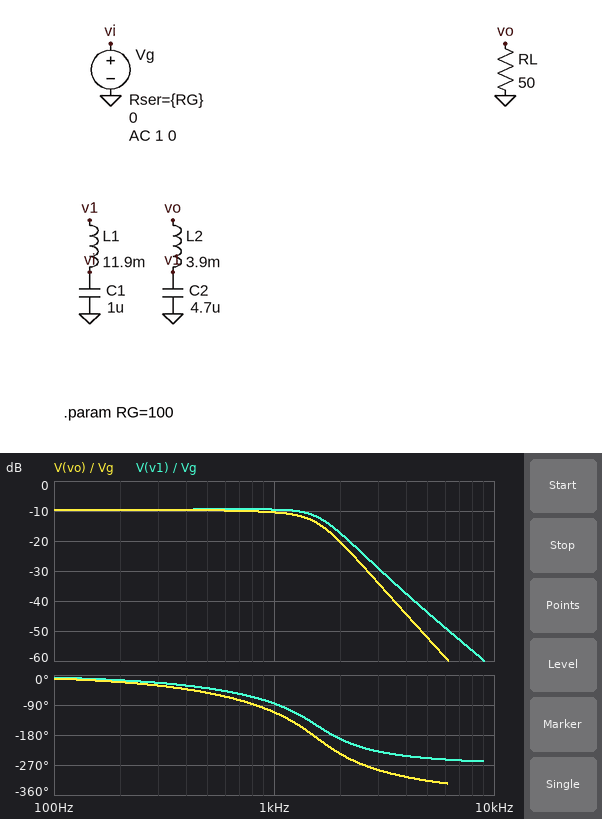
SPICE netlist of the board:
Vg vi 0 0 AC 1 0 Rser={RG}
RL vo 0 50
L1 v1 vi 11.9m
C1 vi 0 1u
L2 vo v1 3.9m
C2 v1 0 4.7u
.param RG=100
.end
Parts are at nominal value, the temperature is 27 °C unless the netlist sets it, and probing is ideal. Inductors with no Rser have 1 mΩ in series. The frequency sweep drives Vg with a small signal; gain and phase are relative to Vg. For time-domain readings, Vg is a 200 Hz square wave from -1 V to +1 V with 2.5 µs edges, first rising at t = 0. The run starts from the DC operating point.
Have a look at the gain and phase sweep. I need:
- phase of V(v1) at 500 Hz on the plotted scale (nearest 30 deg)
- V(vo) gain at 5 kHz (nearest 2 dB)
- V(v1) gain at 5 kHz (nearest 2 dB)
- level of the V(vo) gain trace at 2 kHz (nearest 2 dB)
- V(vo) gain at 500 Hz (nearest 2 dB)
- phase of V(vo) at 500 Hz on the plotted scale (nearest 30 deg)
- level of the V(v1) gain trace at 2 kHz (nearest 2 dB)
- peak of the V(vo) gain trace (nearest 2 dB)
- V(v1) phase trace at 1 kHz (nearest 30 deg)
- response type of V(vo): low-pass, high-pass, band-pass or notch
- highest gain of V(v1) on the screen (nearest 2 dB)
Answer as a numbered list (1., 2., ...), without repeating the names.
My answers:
1. -30 deg
2. -52 dB
3. -44 dB
4. -20 dB
5. -10 dB
6. -60 deg
7. -18 dB
8. -10 dB
9. -90 deg
10. low-pass
11. -10 dB
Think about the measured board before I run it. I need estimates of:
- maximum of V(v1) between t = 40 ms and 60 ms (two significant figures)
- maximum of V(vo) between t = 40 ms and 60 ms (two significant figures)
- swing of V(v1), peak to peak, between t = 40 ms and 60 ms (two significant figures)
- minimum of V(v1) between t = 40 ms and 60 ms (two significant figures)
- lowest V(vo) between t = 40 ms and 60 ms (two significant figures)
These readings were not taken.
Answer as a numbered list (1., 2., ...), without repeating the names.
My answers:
1. 410 mV
2. 380 mV
3. 820 mV
4. -410 mV
5. -380 mV
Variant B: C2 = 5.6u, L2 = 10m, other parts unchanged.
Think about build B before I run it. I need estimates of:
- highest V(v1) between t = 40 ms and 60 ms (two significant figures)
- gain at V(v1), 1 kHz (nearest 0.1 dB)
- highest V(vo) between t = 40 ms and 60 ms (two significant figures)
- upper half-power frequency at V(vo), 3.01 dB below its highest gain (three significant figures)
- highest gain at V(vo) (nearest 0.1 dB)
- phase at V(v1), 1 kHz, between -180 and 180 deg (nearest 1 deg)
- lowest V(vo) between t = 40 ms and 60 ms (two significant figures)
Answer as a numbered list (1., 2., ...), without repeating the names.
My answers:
1. 500 mV
2. -8.3 dB
3. 390 mV
4. 996 Hz
5. -9.4 dB
6. -101 deg
7. -390 mV
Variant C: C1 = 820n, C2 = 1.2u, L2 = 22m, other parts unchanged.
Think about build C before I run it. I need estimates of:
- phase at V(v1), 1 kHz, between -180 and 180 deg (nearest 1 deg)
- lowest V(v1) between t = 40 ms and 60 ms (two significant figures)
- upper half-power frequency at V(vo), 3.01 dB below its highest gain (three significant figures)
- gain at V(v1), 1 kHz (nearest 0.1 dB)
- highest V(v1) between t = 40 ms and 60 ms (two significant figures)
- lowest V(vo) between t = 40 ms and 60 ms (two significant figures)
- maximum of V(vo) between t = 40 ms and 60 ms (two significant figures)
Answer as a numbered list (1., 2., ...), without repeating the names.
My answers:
1. -36 deg
2. -1.1 V
3. 1.28 kHz
4. -2.3 dB
5. 1.1 V
6. -360 mV
7. 360 mV
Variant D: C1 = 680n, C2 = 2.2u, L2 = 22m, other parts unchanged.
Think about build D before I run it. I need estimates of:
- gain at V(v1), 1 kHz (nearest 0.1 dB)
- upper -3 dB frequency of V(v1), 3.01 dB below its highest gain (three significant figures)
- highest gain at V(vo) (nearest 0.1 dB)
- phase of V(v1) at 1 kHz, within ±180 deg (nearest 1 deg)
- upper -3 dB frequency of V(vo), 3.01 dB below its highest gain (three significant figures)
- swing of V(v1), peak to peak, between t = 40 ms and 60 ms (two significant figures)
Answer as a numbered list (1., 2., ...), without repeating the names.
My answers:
1. -2.0 dB
2. 1.70 kHz
3. -9.4 dB
4. -61 deg
5. 1.15 kHz
6. 1.9 V
